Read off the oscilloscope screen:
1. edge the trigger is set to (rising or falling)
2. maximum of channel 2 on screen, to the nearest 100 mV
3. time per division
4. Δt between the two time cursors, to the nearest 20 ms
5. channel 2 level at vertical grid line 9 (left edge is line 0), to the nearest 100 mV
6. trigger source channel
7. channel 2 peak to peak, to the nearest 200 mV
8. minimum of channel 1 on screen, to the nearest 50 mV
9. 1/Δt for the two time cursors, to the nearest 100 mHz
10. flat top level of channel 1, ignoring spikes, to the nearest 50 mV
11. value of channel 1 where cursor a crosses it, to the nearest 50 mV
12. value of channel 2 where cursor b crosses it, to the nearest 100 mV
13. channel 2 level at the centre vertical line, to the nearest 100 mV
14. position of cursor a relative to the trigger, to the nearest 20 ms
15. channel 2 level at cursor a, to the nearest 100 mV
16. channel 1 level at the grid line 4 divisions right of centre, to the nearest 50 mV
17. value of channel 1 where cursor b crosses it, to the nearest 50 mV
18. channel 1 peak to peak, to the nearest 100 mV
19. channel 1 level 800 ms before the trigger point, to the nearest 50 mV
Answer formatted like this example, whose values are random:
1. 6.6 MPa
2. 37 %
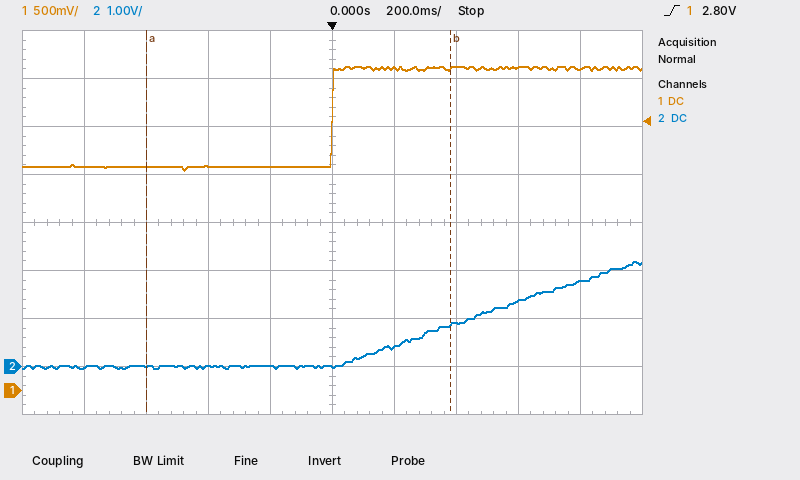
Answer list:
1. rising
2. 2.2 V
3. 200 ms
4. 980 ms
5. 1.8 V
6. channel 1
7. 2.2 V
8. 2.30 V
9. 1.0 Hz
10. 3.35 V
11. 2.35 V
12. 900 mV
13. 0.0 V
14. -600 ms
15. 0.0 V
16. 3.35 V
17. 3.35 V
18. 1.10 V
19. 2.35 V
